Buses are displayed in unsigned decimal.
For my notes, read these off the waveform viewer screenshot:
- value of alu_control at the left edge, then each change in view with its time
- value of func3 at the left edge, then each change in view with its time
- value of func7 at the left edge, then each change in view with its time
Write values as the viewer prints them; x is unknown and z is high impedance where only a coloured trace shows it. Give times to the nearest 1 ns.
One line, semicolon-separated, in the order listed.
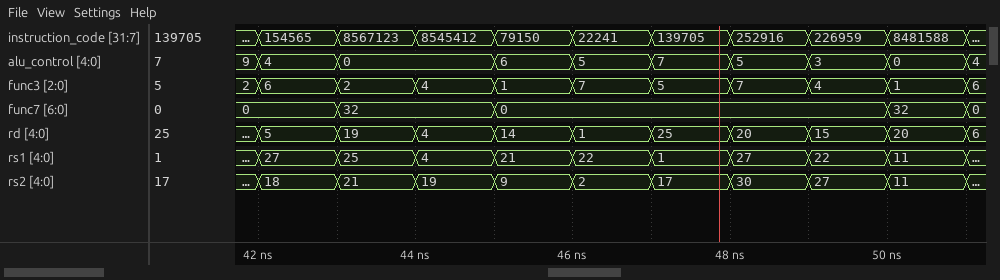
9, 4 at 42 ns, 0 at 43 ns, 6 at 45 ns, 5 at 46 ns, 7 at 47 ns, 5 at 48 ns, 3 at 49 ns, 0 at 50 ns, 4 at 51 ns; 2, 6 at 42 ns, 2 at 43 ns, 4 at 44 ns, 1 at 45 ns, 7 at 46 ns, 5 at 47 ns, 7 at 48 ns, 4 at 49 ns, 1 at 50 ns, 6 at 51 ns; 0, 32 at 43 ns, 0 at 45 ns, 32 at 50 ns, 0 at 51 ns
